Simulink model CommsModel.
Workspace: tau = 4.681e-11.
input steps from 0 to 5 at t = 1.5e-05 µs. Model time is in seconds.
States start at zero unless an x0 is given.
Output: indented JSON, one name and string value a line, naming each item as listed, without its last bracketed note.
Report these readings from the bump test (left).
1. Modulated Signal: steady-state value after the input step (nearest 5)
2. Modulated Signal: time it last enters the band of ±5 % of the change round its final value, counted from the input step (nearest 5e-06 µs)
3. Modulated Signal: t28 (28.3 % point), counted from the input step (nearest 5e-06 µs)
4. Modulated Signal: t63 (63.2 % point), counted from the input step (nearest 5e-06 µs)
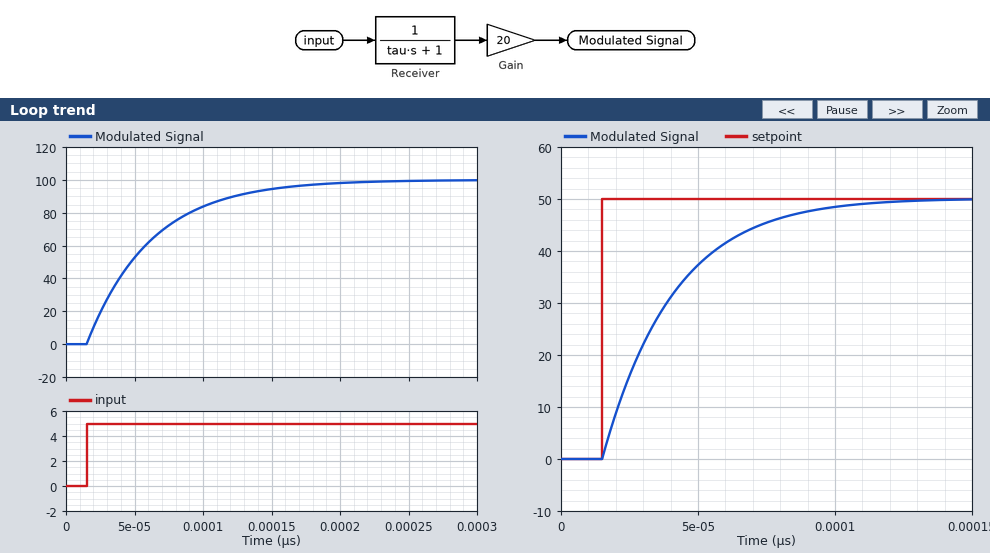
{
  "Modulated Signal: steady-state value after the input step": "100",
  "Modulated Signal: time it last enters the band of ±5 % of the change round its final value, counted from the input step": "0.000140 µs",
  "Modulated Signal: t28 (28.3 % point), counted from the input step": "0.000015 µs",
  "Modulated Signal: t63 (63.2 % point), counted from the input step": "0.000045 µs"
}
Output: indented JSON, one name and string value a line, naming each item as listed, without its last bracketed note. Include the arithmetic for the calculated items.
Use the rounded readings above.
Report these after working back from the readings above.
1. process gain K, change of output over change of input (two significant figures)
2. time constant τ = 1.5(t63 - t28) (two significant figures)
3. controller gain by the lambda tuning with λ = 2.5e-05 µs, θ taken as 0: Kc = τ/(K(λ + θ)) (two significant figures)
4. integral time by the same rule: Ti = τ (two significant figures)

{
  "process gain K, change of output over change of input": "(100 - 0) / 5 = 20",
  "time constant τ = 1.5(t63 - t28)": "1.5 × (4.5e-05 - 1.5e-05) = 0.000045 µs",
  "controller gain by the lambda tuning with λ = 2.5e-05 µs, θ taken as 0: Kc = τ/(K(λ + θ))": "4.5e-05 / (20 × (2.5e-05 + 0)) = 0.090",
  "integral time by the same rule: Ti = τ": "0.000045 µs"
}
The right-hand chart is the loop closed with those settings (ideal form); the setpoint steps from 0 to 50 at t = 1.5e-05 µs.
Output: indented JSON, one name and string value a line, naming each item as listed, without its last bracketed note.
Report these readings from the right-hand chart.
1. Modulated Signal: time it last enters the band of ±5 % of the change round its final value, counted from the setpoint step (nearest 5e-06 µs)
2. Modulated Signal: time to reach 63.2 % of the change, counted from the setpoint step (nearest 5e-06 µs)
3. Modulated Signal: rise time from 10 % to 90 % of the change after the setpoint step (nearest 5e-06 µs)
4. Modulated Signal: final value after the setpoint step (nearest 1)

{
  "Modulated Signal: time it last enters the band of ±5 % of the change round its final value, counted from the setpoint step": "0.000075 µs",
  "Modulated Signal: time to reach 63.2 % of the change, counted from the setpoint step": "0.000025 µs",
  "Modulated Signal: rise time from 10 % to 90 % of the change after the setpoint step": "0.000055 µs",
  "Modulated Signal: final value after the setpoint step": "50"
}
